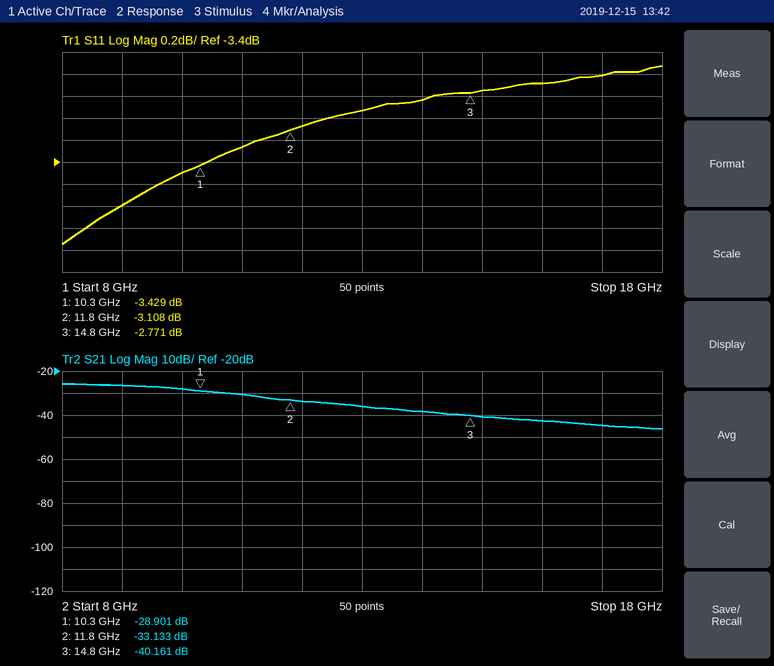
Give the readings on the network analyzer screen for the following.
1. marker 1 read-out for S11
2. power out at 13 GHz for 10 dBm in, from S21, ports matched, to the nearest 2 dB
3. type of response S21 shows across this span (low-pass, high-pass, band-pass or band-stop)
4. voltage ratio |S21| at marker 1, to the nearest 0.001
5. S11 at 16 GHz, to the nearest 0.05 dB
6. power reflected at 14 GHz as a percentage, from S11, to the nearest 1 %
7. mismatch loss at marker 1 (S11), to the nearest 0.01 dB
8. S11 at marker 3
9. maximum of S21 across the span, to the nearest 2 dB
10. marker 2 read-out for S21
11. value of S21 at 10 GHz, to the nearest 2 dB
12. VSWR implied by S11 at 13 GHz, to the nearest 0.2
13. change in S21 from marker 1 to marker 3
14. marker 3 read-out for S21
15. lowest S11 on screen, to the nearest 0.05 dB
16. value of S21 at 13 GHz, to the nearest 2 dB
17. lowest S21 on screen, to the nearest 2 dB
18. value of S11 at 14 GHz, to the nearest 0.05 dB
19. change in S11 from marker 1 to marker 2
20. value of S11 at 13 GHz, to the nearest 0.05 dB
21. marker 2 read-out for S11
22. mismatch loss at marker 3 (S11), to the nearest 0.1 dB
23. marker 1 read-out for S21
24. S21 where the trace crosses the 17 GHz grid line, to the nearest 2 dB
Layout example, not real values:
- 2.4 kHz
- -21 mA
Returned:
- -3.429 dB
- -26 dBm
- low-pass
- 0.036
- -2.70 dB
- 52 %
- 2.63 dB
- -2.771 dB
- -26 dB
- -33.133 dB
- -28 dB
- 6.0
- -11.260 dB
- -40.161 dB
- -4.15 dB
- -36 dB
- -46 dB
- -2.85 dB
- 0.321 dB
- -2.95 dB
- -3.108 dB
- 3.3 dB
- -28.901 dB
- -44 dB
